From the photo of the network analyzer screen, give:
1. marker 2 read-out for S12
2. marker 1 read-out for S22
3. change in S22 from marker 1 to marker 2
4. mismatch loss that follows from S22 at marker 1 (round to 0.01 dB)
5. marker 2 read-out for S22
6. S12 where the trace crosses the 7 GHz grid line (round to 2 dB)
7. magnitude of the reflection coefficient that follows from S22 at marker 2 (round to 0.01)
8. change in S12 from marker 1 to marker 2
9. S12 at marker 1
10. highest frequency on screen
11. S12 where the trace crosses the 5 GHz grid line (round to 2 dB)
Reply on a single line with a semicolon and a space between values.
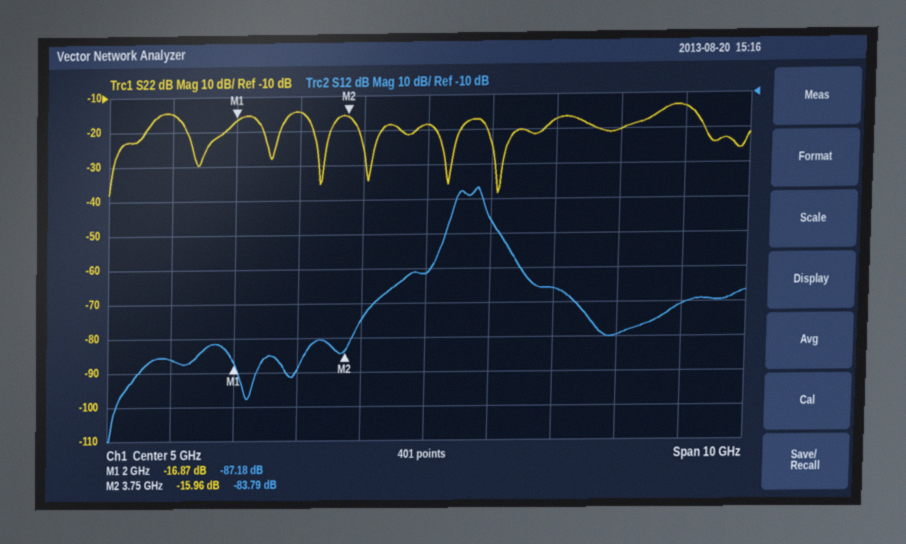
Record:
-83.79 dB; -16.87 dB; 0.91 dB; 0.09 dB; -15.96 dB; -66 dB; 0.16; 3.39 dB; -87.18 dB; 10 GHz; -62 dB
